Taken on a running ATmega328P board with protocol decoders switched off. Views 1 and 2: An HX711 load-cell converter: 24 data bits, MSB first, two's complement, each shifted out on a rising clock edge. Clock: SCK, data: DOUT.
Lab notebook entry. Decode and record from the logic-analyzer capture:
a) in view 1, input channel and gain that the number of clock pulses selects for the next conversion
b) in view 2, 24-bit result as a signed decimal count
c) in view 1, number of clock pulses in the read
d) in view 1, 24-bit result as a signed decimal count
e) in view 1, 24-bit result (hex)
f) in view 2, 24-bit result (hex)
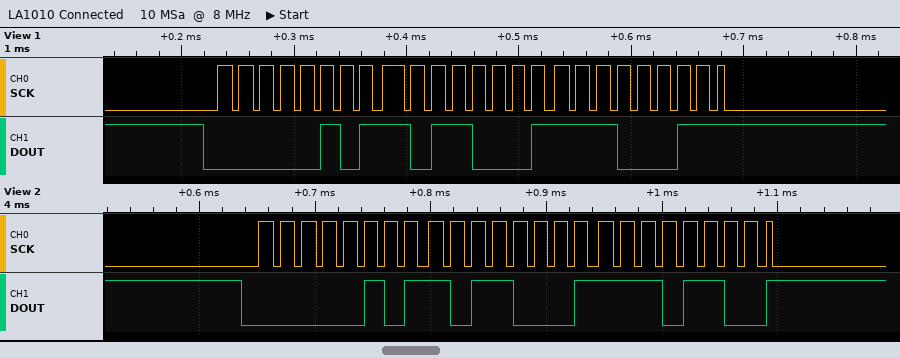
channel A, gain 128
373228
25
373219
0x05B1E3
0x05B1EC
